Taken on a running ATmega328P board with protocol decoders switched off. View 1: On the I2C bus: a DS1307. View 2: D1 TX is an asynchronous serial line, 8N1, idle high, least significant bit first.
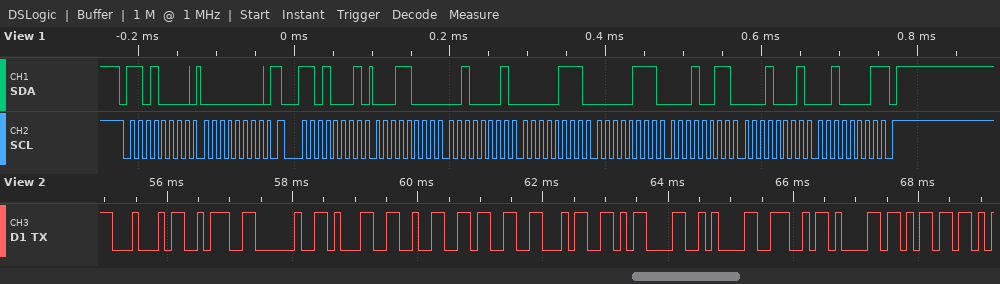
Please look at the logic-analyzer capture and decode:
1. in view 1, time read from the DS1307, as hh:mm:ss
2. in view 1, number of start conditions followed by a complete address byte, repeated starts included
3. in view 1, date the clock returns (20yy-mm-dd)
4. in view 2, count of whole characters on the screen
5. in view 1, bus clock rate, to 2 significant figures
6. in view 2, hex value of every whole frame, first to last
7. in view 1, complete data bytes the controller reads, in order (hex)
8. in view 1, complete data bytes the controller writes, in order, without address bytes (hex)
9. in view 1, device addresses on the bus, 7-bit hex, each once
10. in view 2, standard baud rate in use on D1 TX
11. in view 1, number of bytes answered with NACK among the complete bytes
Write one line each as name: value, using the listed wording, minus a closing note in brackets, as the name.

in view 1, time read from the DS1307, as hh:mm:ss: 07:21:18
in view 1, number of start conditions followed by a complete address byte, repeated starts included: 2
in view 1, date the clock returns: 2021-11-13
in view 2, count of whole characters on the screen: 12
in view 1, bus clock rate, to 2 significant figures: 100 kHz
in view 2, hex value of every whole frame, first to last: 44 3A 20 31 32 33 34 0D 0A 4E 61 6D
in view 1, complete data bytes the controller reads, in order: 18 21 07 07 13 11 21
in view 1, complete data bytes the controller writes, in order, without address bytes: 00
in view 1, device addresses on the bus, 7-bit hex, each once: 0x68
in view 2, standard baud rate in use on D1 TX: 9600 baud
in view 1, number of bytes answered with NACK among the complete bytes: 1
